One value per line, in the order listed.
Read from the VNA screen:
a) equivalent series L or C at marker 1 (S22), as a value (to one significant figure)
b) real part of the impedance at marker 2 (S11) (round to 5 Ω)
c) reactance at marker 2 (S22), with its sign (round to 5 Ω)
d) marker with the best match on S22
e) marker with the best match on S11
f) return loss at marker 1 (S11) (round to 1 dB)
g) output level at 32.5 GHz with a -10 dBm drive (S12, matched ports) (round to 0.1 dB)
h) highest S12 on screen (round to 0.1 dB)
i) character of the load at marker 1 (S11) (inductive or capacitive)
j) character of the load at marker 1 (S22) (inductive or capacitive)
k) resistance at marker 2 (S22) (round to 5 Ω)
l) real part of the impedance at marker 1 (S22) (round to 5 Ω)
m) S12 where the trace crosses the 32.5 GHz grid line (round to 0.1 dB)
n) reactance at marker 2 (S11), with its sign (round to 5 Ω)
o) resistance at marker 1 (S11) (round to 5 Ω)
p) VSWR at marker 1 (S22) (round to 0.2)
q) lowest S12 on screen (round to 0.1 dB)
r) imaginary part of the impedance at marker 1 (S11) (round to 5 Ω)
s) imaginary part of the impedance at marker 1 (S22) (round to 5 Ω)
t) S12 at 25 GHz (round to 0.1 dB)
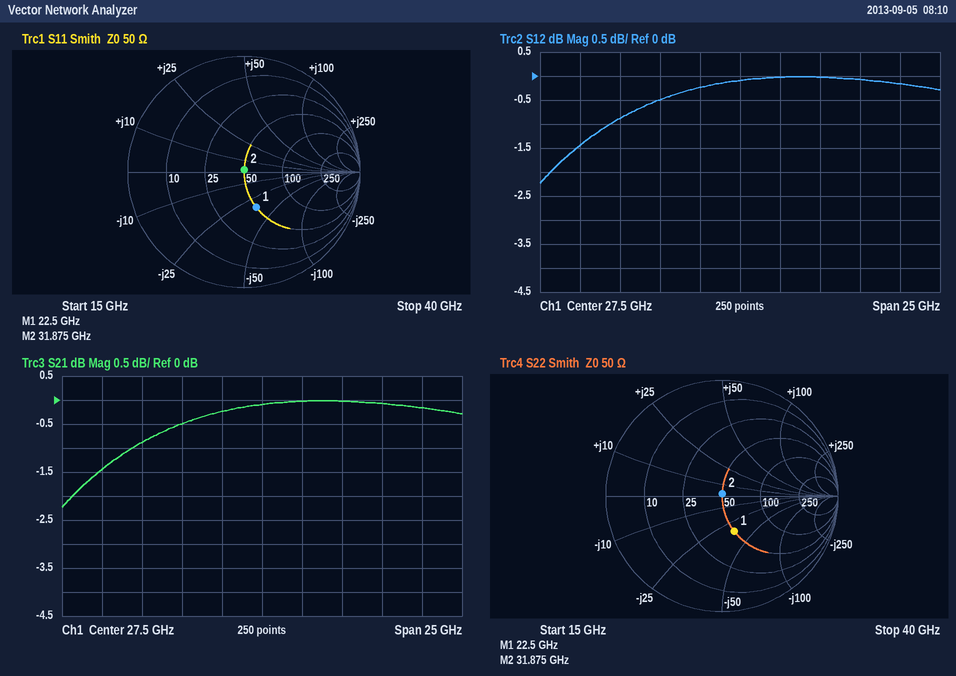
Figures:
200 fF
50 Ω
0 Ω
marker 2
marker 2
10 dB
-10.0 dBm
0.0 dB
capacitive
capacitive
50 Ω
50 Ω
0.0 dB
0 Ω
50 Ω
2.0
-2.2 dB
-35 Ω
-35 Ω
-0.2 dB
